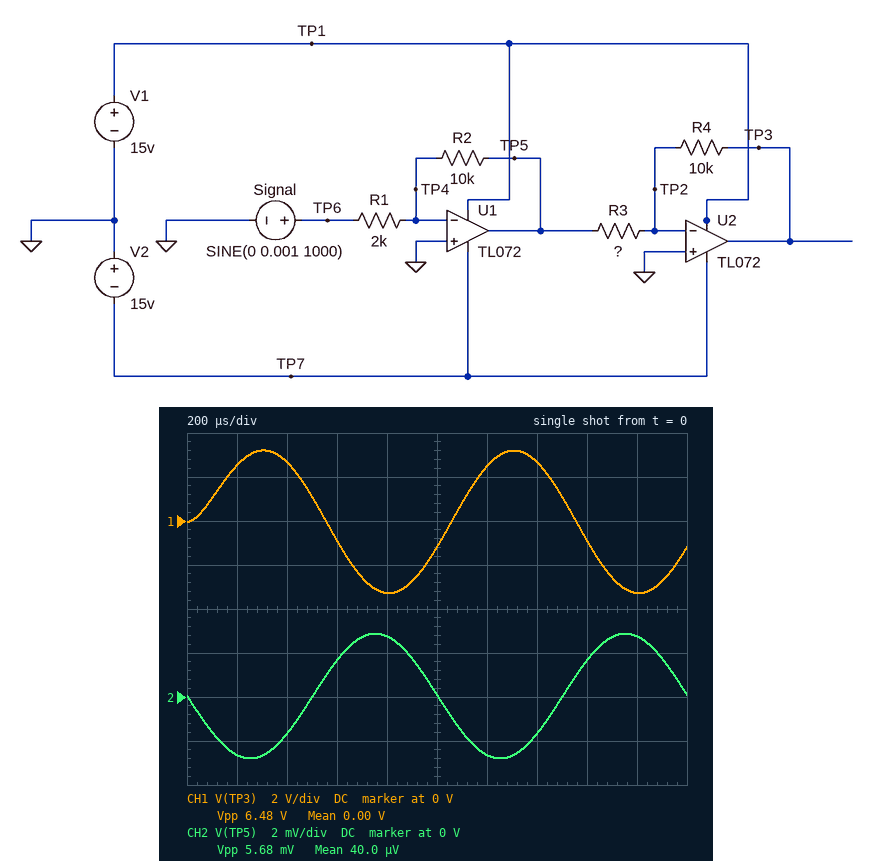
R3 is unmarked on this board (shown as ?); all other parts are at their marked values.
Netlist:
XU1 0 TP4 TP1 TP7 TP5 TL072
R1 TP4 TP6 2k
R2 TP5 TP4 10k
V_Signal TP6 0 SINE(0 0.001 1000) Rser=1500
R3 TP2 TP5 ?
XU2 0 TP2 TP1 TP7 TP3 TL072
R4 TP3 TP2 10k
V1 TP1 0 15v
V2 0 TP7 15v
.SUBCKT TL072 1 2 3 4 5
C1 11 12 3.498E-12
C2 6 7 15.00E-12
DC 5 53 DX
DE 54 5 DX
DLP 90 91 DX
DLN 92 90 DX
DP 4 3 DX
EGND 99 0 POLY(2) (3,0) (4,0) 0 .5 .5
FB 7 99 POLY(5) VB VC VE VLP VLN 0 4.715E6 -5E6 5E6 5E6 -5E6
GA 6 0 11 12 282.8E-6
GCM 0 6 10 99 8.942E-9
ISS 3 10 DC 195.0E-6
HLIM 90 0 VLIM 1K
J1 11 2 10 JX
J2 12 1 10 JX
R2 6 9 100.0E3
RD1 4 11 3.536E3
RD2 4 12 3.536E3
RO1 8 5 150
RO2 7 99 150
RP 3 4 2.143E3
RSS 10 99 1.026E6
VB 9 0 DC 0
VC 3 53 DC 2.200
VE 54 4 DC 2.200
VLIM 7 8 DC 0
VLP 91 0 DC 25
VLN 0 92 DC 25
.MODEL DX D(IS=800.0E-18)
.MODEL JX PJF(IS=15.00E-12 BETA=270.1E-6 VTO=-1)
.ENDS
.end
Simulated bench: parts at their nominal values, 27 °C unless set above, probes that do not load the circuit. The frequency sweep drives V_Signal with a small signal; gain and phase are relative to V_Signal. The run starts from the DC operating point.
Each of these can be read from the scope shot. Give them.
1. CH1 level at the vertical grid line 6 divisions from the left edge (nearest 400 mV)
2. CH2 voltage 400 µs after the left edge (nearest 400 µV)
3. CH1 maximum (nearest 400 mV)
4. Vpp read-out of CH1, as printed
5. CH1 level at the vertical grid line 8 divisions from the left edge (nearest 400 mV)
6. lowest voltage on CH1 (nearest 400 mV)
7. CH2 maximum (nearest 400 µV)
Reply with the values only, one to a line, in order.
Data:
2.4 V
-1.6 mV
3.2 V
6.48 V
-800 mV
-3.2 V
2.8 mV
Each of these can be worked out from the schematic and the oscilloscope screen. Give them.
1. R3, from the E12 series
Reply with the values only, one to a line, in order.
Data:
8.2 Ω
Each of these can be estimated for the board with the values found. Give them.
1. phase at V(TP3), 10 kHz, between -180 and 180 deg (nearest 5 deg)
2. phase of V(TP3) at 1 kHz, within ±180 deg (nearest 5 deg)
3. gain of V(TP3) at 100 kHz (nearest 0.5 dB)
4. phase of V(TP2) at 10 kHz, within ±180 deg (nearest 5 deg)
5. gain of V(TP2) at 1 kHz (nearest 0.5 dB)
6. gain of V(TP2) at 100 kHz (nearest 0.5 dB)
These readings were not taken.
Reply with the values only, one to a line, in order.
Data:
-75 deg
-20 deg
39.0 dB
-165 deg
-0.5 dB
8.5 dB
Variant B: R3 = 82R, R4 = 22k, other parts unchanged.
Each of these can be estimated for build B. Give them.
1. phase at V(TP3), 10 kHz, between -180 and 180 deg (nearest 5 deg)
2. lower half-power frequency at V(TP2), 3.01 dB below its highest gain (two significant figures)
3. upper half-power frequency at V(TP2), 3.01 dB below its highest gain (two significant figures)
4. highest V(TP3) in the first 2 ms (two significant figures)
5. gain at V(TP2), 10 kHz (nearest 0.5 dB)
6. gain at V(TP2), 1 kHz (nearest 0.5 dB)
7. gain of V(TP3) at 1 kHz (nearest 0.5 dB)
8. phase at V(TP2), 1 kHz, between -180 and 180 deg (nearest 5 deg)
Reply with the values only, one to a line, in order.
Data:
-40 deg
12 kHz
1.1 MHz
750 mV
5.0 dB
-13.0 dB
57.5 dB
-95 deg
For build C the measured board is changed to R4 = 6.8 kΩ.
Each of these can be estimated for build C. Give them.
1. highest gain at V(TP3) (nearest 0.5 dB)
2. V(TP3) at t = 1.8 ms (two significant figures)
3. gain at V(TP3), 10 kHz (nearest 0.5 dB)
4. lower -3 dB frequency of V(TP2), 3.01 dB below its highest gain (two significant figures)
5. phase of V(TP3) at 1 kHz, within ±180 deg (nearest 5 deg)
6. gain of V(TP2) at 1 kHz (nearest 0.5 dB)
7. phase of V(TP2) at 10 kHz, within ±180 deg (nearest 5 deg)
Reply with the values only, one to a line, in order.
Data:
67.5 dB
-2.3 V
58.5 dB
3.7 kHz
-15 deg
-3.5 dB
-160 deg
